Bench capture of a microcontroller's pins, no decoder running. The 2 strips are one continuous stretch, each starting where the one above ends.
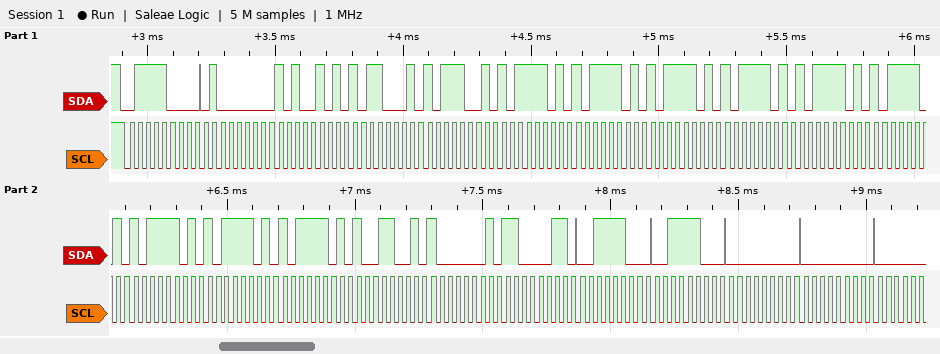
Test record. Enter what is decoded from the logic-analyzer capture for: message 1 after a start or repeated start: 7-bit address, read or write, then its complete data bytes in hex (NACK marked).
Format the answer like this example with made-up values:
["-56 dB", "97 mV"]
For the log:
["0x3C write: 40 A5 B1 B9 BD BD BD BD BD BD BD BD BD 99 81 C3 3C 3C 00 00"]
